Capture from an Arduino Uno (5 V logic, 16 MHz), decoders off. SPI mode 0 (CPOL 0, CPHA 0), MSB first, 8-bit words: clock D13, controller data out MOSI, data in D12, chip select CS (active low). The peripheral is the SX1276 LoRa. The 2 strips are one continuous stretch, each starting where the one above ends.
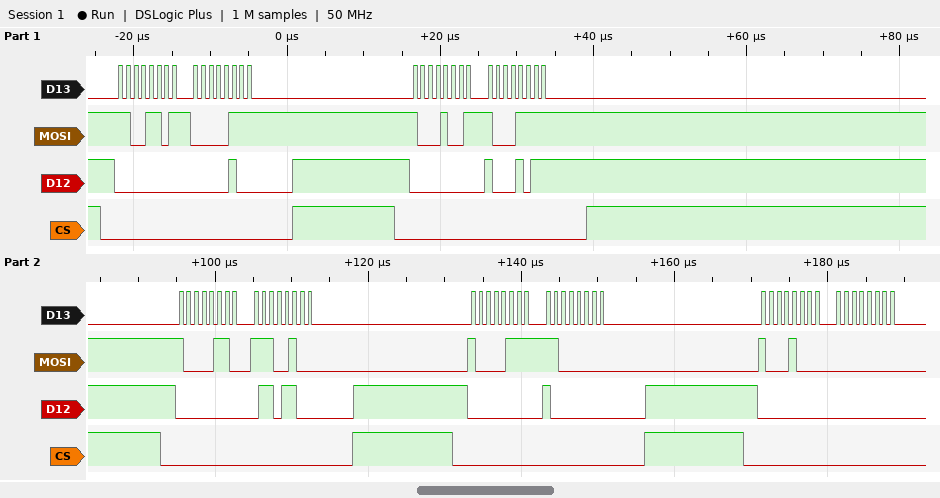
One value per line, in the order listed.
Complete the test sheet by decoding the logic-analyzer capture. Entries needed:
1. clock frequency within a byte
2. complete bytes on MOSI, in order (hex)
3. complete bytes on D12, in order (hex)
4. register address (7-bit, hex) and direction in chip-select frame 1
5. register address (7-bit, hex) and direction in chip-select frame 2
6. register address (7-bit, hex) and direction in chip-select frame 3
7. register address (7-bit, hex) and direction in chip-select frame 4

1 MHz
CD 07 89 8F 86 E4 87 C0 88 00
00 04 00 8B 00 6C 00 80 00 00
0x4D write
0x09 write
0x06 write
0x07 write
